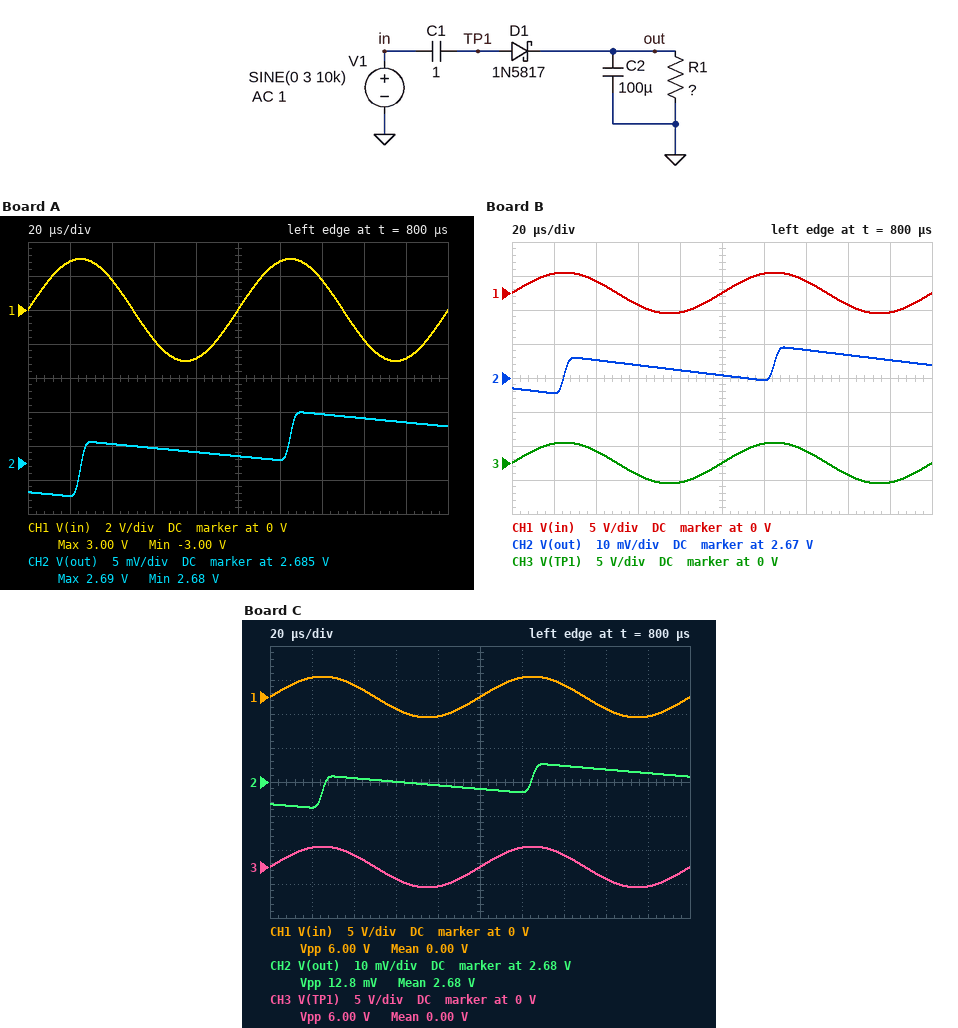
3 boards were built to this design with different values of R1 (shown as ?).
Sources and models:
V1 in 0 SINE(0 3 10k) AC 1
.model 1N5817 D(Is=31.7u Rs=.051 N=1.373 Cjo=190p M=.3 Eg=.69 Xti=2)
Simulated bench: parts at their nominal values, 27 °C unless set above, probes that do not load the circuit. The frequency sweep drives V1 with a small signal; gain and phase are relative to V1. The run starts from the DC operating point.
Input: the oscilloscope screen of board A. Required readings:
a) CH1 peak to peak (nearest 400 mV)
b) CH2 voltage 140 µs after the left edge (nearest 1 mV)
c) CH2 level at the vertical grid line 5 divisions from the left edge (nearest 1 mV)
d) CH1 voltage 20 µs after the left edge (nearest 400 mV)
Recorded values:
6.0 V
2.692 V
2.686 V
2.8 V
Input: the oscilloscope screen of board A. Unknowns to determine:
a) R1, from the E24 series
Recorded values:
910 Ω
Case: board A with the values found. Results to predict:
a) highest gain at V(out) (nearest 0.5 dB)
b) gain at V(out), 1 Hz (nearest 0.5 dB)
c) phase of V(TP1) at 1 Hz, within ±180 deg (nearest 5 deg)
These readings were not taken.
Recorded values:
-7.0 dB
-7.5 dB
0 deg
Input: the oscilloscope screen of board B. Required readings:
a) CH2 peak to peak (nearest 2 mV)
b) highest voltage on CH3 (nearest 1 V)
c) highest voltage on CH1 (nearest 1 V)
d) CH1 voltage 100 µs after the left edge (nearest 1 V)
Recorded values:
14 mV
3 V
3 V
0 V
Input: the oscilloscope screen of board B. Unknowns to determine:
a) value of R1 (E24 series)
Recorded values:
360 Ω
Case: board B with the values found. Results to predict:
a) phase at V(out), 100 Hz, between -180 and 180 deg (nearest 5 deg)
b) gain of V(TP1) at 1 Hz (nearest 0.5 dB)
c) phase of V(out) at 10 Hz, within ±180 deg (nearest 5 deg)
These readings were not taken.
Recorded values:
-85 deg
0 dB
-60 deg
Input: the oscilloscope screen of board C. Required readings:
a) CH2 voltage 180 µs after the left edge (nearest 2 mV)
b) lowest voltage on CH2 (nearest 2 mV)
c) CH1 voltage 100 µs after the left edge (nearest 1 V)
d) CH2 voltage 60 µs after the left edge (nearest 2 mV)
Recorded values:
2.682 V
2.672 V
0 V
2.680 V
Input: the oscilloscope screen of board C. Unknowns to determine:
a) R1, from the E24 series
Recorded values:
510 Ω
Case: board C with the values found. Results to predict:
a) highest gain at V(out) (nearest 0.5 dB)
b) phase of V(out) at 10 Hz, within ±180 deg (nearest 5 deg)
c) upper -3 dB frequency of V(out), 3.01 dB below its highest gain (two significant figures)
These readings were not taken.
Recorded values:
-10.0 dB
-65 deg
4.5 Hz
